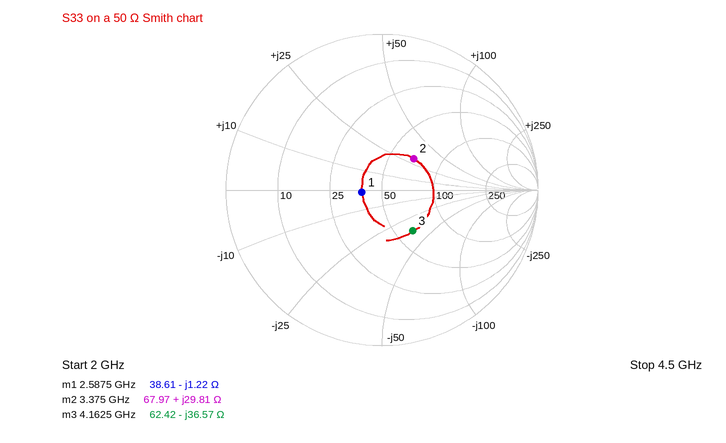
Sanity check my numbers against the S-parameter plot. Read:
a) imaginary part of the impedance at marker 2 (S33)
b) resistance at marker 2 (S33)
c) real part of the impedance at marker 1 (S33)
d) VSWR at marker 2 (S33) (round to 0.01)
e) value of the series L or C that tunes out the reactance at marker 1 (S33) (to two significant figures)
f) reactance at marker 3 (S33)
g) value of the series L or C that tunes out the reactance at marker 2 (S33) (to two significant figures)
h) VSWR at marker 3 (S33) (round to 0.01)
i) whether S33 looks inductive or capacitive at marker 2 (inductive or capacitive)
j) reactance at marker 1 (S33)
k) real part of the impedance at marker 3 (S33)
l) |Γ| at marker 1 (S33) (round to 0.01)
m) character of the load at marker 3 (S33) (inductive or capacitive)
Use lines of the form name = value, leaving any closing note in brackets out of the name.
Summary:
imaginary part of the impedance at marker 2 = +29.81 Ω
resistance at marker 2 = 67.97 Ω
real part of the impedance at marker 1 = 38.61 Ω
VSWR at marker 2 (S33) = 1.80
value of the series L or C that tunes out the reactance at marker 1 (S33) = 75 pH
reactance at marker 3 = -36.57 Ω
value of the series L or C that tunes out the reactance at marker 2 (S33) = 1.6 pF
VSWR at marker 3 (S33) = 1.97
whether S33 looks inductive or capacitive at marker 2 = inductive
reactance at marker 1 = -1.22 Ω
real part of the impedance at marker 3 = 62.42 Ω
|Γ| at marker 1 (S33) = 0.13
character of the load at marker 3 (S33) = capacitive
